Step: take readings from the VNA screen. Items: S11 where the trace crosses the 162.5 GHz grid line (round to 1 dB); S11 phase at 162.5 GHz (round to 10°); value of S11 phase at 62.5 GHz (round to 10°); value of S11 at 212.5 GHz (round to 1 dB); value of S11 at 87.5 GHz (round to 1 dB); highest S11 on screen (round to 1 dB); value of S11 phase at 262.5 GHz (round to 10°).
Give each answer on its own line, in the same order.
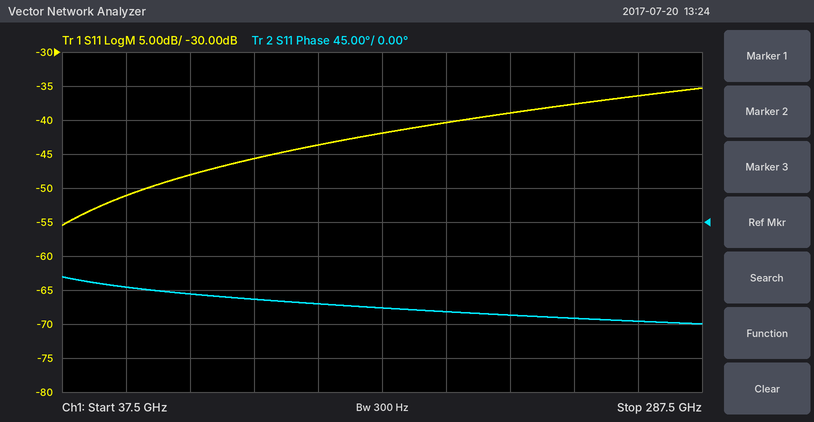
-42 dB
-110°
-90°
-39 dB
-48 dB
-35 dB
-130°
